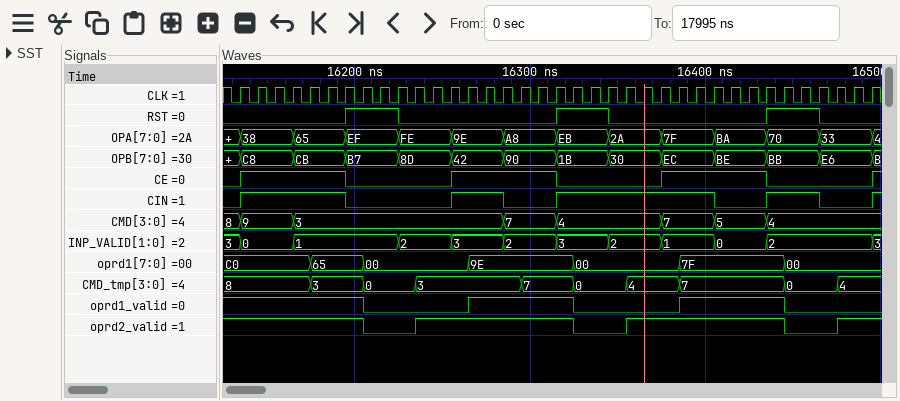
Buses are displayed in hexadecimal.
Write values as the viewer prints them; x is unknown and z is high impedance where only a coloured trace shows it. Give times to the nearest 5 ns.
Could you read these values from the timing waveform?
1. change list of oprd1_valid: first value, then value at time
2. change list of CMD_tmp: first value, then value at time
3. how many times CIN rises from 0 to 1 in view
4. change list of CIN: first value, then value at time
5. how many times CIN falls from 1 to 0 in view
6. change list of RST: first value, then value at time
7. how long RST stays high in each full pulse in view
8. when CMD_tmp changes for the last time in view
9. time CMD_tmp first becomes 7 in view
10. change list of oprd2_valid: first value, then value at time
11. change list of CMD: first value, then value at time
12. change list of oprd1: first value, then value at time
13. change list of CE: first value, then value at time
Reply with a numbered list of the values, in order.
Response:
1. 1, 0 at 16205 ns, 1 at 16265 ns, 0 at 16325 ns, 1 at 16385 ns, 0 at 16445 ns
2. 8, 3 at 16175 ns, 0 at 16205 ns, 3 at 16235 ns, 7 at 16295 ns, 0 at 16325 ns, 4 at 16355 ns, 7 at 16385 ns, 0 at 16445 ns, 4 at 16475 ns
3. 5
4. 0, 1 at 16135 ns, 0 at 16195 ns, 1 at 16255 ns, 0 at 16285 ns, 1 at 16315 ns, 0 at 16405 ns, 1 at 16435 ns, 0 at 16465 ns, 1 at 16495 ns
5. 4
6. 0, 1 at 16195 ns, 0 at 16225 ns, 1 at 16315 ns, 0 at 16345 ns, 1 at 16435 ns, 0 at 16465 ns
7. 30 ns, 30 ns, 30 ns
8. 16475 ns
9. 16295 ns
10. 1, 0 at 16205 ns, 1 at 16235 ns, 0 at 16325 ns, 1 at 16355 ns, 0 at 16445 ns, 1 at 16475 ns
11. 8, 9 at 16135 ns, 3 at 16165 ns, 7 at 16285 ns, 4 at 16315 ns, 7 at 16375 ns, 5 at 16405 ns, 4 at 16435 ns
12. C0, 65 at 16175 ns, 00 at 16205 ns, 9E at 16265 ns, 00 at 16325 ns, 7F at 16385 ns, 00 at 16445 ns
13. 0, 1 at 16135 ns, 0 at 16195 ns, 1 at 16255 ns, 0 at 16315 ns, 1 at 16375 ns, 0 at 16435 ns, 1 at 16495 ns
